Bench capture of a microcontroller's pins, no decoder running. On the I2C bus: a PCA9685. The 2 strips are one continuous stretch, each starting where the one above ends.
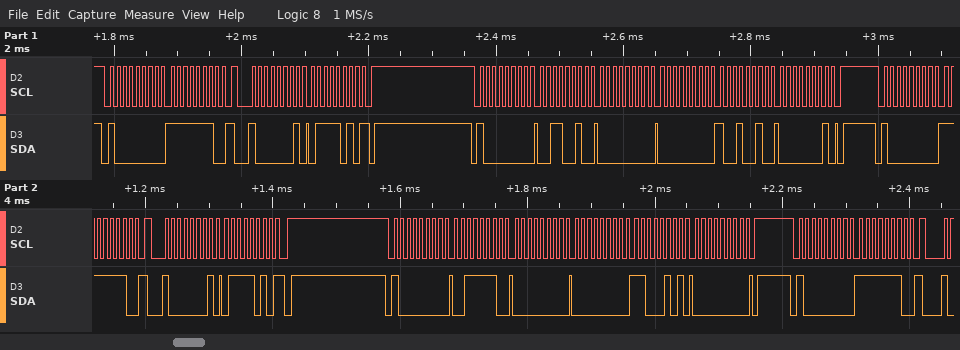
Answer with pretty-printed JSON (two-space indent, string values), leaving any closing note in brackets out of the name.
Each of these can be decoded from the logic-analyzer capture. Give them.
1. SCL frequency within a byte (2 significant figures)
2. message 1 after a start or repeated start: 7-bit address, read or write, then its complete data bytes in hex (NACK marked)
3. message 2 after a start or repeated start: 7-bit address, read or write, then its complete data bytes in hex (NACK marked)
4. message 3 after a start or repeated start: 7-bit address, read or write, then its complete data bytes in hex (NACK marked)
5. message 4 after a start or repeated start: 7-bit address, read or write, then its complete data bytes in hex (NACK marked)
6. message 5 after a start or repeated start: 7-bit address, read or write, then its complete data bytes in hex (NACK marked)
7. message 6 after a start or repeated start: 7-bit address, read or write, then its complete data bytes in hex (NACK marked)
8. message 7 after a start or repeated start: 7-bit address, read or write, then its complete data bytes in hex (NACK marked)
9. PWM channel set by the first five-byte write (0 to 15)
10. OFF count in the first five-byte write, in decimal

{
  "SCL frequency within a byte": "100 kHz",
  "message 1 after a start or repeated start: 7-bit address, read or write, then its complete data bytes in hex": "0x40 write: FE",
  "message 2 after a start or repeated start: 7-bit address, read or write, then its complete data bytes in hex": "0x40 read: 7A NACK",
  "message 3 after a start or repeated start: 7-bit address, read or write, then its complete data bytes in hex": "0x40 write: 32 00 00 92 01",
  "message 4 after a start or repeated start: 7-bit address, read or write, then its complete data bytes in hex": "0x40 write: FE",
  "message 5 after a start or repeated start: 7-bit address, read or write, then its complete data bytes in hex": "0x40 read: 7A NACK",
  "message 6 after a start or repeated start: 7-bit address, read or write, then its complete data bytes in hex": "0x40 write: 3E 00 00 C5 00",
  "message 7 after a start or repeated start: 7-bit address, read or write, then its complete data bytes in hex": "0x40 write: FE",
  "PWM channel set by the first five-byte write": "11",
  "OFF count in the first five-byte write, in decimal": "402"
}
